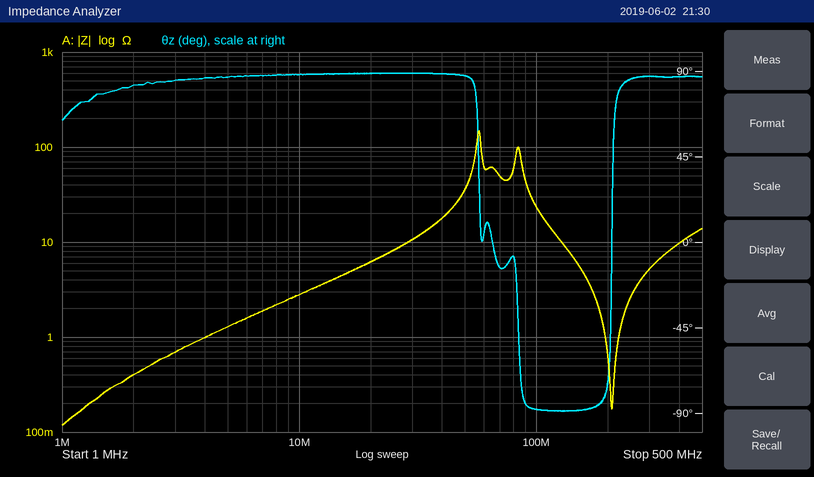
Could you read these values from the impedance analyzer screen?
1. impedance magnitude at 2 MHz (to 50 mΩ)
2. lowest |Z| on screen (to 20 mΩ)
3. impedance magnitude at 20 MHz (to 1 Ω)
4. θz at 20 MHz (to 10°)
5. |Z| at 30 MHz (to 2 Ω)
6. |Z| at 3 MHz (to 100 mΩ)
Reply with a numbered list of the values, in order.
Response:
1. 400 mΩ
2. 120 mΩ
3. 6 Ω
4. 90°
5. 10 Ω
6. 700 mΩ
